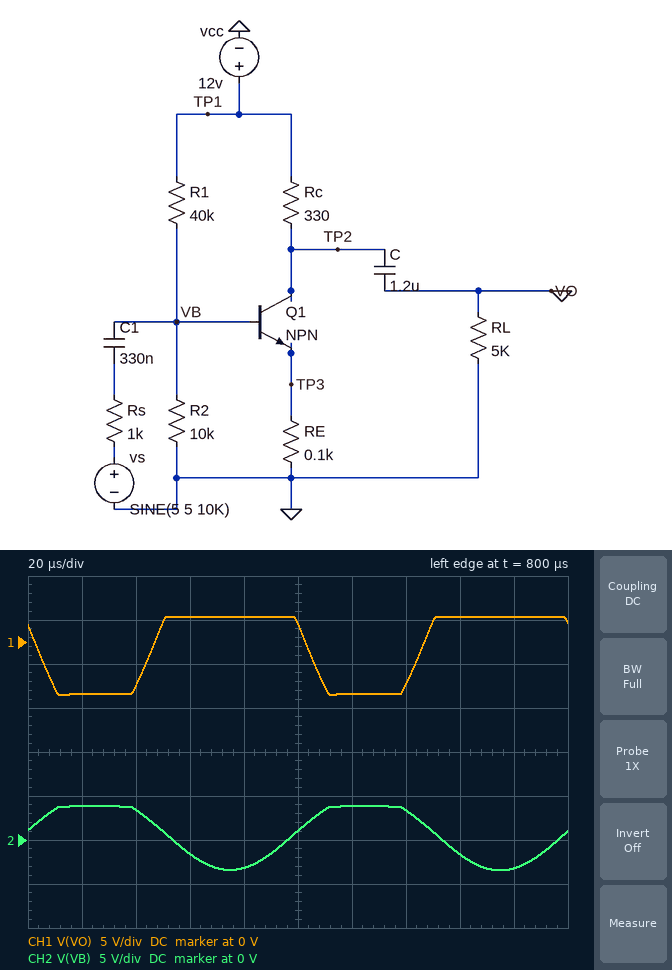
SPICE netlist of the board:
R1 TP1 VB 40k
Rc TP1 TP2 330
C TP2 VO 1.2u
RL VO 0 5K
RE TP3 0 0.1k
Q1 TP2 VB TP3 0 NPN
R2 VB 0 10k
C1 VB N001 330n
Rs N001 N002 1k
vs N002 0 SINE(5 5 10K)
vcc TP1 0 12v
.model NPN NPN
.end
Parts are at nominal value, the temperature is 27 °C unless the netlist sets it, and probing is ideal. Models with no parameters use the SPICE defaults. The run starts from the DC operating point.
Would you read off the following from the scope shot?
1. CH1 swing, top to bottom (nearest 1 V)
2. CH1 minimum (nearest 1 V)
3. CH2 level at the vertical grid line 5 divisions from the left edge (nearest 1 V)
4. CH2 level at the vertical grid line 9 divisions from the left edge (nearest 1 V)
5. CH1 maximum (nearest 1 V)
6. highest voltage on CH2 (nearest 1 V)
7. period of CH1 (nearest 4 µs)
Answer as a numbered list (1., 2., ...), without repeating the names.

1. 9 V
2. -6 V
3. 1 V
4. -3 V
5. 3 V
6. 4 V
7. 100 µs
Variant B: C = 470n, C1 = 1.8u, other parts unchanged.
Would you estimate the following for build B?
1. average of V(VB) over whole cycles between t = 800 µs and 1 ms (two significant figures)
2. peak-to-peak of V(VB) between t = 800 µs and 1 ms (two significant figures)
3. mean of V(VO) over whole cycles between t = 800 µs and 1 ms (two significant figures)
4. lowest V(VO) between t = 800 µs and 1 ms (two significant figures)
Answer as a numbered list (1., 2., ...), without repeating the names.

1. 1.1 V
2. 6.8 V
3. -770 mV
4. -5.8 V
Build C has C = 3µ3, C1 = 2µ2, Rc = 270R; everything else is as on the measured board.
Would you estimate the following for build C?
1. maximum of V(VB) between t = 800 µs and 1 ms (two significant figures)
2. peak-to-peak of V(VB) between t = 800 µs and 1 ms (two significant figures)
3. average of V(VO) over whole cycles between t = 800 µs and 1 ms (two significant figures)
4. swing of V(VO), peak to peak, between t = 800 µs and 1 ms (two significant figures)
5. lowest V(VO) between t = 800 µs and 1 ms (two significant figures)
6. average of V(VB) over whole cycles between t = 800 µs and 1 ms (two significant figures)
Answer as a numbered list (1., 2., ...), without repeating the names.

1. 4.3 V
2. 7.1 V
3. -1.3 V
4. 8.4 V
5. -6.1 V
6. 1.3 V
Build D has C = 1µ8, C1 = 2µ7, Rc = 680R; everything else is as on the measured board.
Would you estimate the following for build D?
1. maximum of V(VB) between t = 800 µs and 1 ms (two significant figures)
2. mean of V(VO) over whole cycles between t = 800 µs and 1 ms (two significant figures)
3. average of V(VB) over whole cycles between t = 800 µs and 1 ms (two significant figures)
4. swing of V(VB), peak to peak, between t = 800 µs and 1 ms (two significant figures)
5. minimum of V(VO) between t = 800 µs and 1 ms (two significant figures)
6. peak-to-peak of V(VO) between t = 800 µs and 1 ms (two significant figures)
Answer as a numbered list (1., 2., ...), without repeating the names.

1. 2.8 V
2. 560 mV
3. 630 mV
4. 5.7 V
5. -4.4 V
6. 9.6 V
